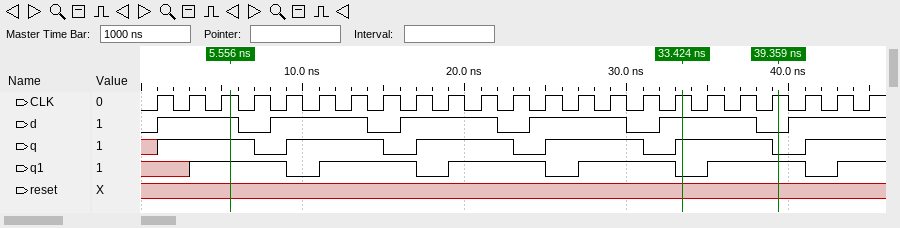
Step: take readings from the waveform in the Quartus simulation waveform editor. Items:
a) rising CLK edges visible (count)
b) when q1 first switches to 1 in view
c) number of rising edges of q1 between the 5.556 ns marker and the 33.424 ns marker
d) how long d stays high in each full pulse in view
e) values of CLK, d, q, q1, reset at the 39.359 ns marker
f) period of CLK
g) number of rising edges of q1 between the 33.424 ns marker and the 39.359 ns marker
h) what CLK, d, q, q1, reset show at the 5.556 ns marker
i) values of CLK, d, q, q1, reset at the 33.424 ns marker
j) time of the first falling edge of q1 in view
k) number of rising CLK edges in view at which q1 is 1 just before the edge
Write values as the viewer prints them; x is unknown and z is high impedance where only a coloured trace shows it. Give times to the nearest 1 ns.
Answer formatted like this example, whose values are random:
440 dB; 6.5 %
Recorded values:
23; 3 ns; 3; 5 ns, 6 ns, 6 ns, 6 ns, 6 ns; CLK=1, d=0, q=0, q1=1, reset=x; 2 ns; 1; CLK=1, d=1, q=1, q1=1, reset=x; CLK=1, d=1, q=1, q1=0, reset=x; 9 ns; 16
